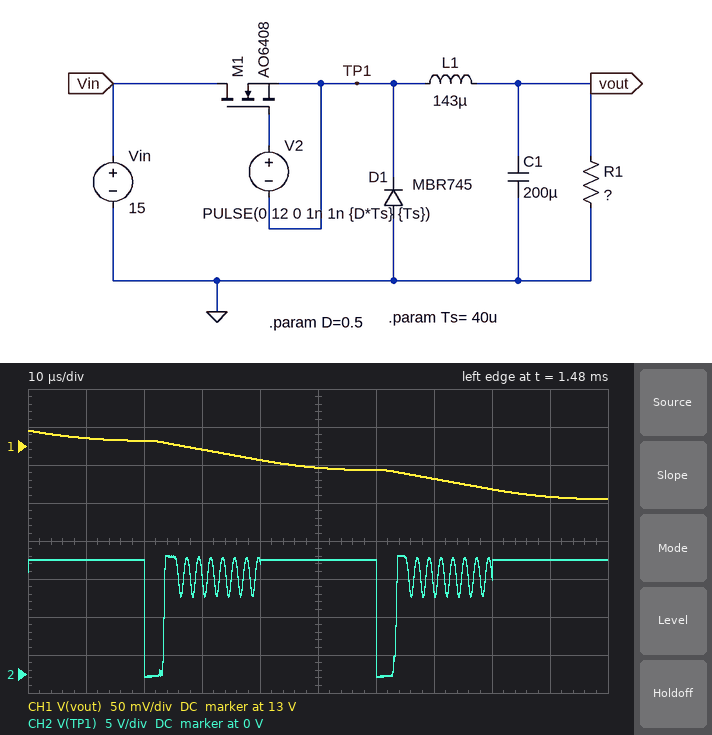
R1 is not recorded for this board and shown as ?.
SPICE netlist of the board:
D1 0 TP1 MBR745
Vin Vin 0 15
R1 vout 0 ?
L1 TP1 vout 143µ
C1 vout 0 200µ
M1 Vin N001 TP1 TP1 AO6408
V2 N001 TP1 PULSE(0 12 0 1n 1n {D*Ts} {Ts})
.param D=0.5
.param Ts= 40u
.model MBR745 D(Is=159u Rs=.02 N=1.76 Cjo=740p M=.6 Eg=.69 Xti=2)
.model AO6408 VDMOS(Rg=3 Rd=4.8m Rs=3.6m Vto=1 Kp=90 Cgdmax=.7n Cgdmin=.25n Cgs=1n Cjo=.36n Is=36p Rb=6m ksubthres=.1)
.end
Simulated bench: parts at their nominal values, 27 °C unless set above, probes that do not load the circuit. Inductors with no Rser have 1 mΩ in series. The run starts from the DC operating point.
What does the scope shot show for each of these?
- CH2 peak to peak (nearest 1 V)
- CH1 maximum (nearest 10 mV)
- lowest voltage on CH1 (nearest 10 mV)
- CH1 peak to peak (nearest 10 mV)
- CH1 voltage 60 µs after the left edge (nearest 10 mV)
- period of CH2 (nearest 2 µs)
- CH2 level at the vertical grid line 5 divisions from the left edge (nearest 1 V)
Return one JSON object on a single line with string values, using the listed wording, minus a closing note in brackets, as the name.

{"CH2 peak to peak": "16 V", "CH1 maximum": "13.02 V", "lowest voltage on CH1": "12.93 V", "CH1 peak to peak": "90 mV", "CH1 voltage 60 µs after the left edge": "12.97 V", "period of CH2": "40 µs", "CH2 level at the vertical grid line 5 divisions from the left edge": "15 V"}
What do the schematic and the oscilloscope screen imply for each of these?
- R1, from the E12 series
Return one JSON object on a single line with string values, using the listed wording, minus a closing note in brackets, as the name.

{"R1, from the E12 series": "47 Ω"}
